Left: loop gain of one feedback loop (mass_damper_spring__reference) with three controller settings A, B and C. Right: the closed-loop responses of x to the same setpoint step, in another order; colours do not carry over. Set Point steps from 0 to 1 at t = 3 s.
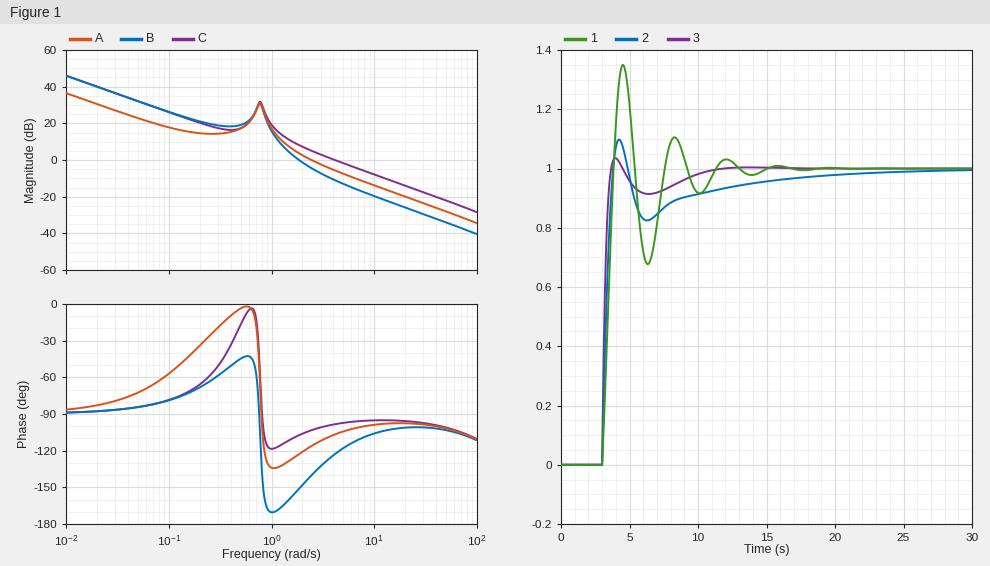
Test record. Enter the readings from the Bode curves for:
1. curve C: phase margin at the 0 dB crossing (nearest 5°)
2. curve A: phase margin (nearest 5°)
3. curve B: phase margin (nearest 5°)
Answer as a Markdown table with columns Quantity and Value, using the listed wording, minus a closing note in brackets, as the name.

| Quantity | Value |
|---|---|
| curve C: phase margin at the 0 dB crossing | 80° |
| curve A: phase margin | 65° |
| curve B: phase margin | 30° |
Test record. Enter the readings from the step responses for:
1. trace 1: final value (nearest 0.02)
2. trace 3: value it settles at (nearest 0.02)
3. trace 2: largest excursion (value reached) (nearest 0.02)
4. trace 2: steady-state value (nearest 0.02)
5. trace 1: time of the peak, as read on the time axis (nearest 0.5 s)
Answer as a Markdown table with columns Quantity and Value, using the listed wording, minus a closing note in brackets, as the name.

| Quantity | Value |
|---|---|
| trace 1: final value | 1.00 |
| trace 3: value it settles at | 1.00 |
| trace 2: largest excursion (value reached) | 1.10 |
| trace 2: steady-state value | 1.00 |
| trace 1: time of the peak, as read on the time axis | 4.5 s |
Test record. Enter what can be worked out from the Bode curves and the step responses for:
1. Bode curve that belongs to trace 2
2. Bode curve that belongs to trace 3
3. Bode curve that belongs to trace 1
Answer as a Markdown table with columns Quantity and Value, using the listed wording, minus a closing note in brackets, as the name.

| Quantity | Value |
|---|---|
| Bode curve that belongs to trace 2 | A |
| Bode curve that belongs to trace 3 | C |
| Bode curve that belongs to trace 1 | B |
